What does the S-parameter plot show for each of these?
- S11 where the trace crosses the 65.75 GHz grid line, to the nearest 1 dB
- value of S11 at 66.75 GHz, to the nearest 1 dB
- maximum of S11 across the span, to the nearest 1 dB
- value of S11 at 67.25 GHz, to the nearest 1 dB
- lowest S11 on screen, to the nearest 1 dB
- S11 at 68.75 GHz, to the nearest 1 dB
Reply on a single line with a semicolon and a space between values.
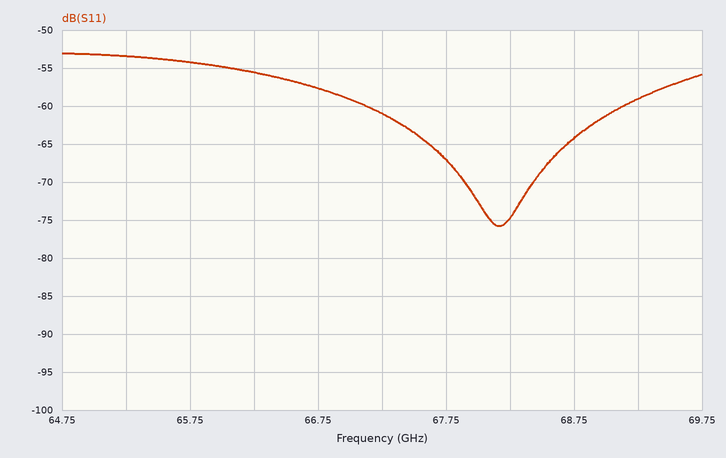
-54 dB; -58 dB; -53 dB; -61 dB; -76 dB; -64 dB
